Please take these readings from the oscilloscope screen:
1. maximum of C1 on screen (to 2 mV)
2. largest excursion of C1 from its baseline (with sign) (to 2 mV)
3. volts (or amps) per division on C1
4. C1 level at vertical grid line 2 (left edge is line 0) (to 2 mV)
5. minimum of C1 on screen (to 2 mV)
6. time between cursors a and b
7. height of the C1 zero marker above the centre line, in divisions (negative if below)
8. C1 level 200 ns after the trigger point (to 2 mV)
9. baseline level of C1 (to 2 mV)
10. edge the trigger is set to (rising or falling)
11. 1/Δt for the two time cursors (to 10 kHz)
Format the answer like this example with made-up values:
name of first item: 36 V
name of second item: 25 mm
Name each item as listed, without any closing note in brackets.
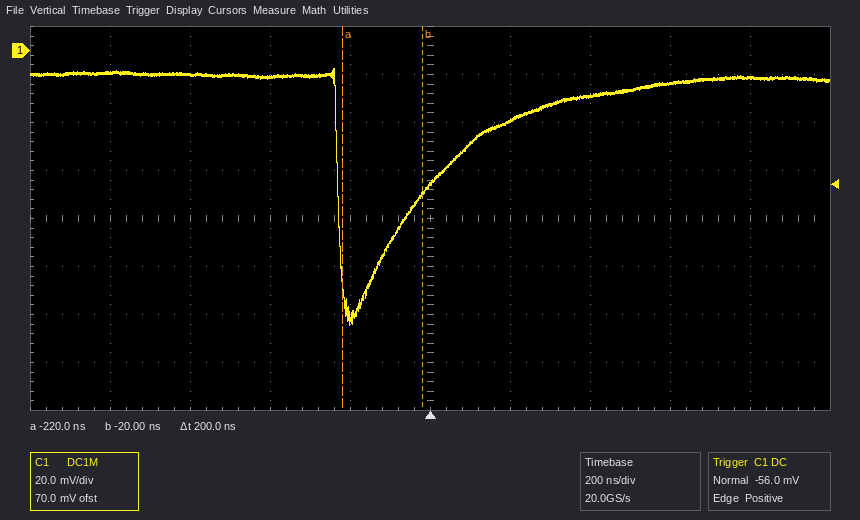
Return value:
maximum of C1 on screen: -8 mV
largest excursion of C1 from its baseline (with sign): -104 mV
volts (or amps) per division on C1: 20 mV
C1 level at vertical grid line 2 (left edge is line 0): -10 mV
minimum of C1 on screen: -114 mV
time between cursors a and b: 200 ns
height of the C1 zero marker above the centre line, in divisions: +3.5 div
C1 level 200 ns after the trigger point: -30 mV
baseline level of C1: -10 mV
edge the trigger is set to: rising
1/Δt for the two time cursors: 5.00 MHz
